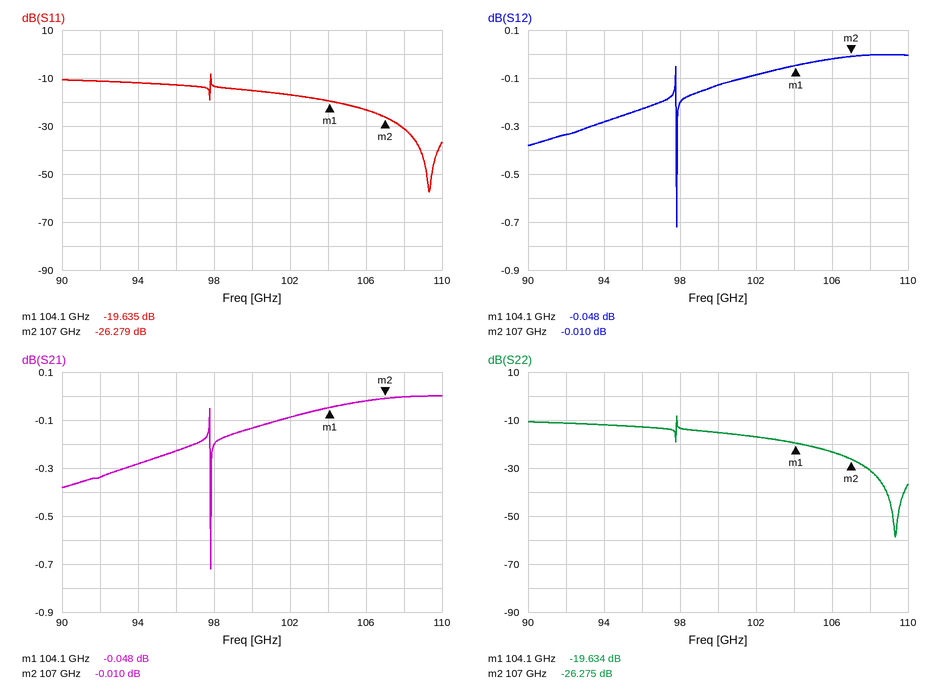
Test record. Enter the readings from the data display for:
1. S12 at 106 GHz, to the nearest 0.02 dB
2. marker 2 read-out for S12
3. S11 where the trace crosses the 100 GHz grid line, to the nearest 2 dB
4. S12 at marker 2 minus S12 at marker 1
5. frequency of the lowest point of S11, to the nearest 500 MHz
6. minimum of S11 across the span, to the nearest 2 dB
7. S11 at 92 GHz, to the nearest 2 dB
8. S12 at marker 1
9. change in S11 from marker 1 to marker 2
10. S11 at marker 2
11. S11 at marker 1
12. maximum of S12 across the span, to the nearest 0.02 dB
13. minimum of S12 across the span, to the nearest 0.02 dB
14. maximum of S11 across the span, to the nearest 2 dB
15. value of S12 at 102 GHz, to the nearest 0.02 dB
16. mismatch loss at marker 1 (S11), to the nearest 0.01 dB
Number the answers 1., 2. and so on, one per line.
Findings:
1. -0.02 dB
2. -0.010 dB
3. -16 dB
4. 0.038 dB
5. 109.5 GHz
6. -58 dB
7. -12 dB
8. -0.048 dB
9. -6.644 dB
10. -26.279 dB
11. -19.635 dB
12. 0.00 dB
13. -0.72 dB
14. -8 dB
15. -0.08 dB
16. 0.05 dB
